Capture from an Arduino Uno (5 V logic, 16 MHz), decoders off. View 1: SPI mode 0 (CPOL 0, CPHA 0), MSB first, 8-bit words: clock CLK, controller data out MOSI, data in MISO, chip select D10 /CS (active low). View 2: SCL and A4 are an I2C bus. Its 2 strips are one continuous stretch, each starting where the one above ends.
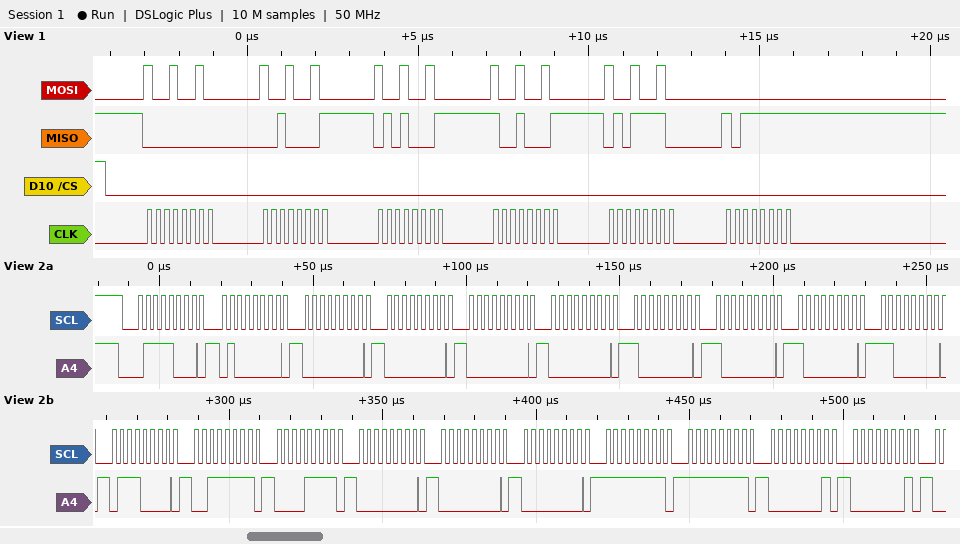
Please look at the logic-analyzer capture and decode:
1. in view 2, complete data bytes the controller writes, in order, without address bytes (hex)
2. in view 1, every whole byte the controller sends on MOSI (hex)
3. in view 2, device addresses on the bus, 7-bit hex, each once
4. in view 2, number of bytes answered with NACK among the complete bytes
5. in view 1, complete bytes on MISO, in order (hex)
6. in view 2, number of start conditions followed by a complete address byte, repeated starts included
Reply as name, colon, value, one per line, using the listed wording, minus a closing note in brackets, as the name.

in view 2, complete data bytes the controller writes, in order, without address bytes: 40 00 00 00 00 80 80 80 C0 70 3F 0F 00 00 00 FF FF 01 01
in view 1, every whole byte the controller sends on MOSI: 92 92 92 92 92 00
in view 2, device addresses on the bus, 7-bit hex, each once: 0x3C
in view 2, number of bytes answered with NACK among the complete bytes: 0
in view 1, complete bytes on MISO, in order: 00 21 51 91 5E BF
in view 2, number of start conditions followed by a complete address byte, repeated starts included: 1
